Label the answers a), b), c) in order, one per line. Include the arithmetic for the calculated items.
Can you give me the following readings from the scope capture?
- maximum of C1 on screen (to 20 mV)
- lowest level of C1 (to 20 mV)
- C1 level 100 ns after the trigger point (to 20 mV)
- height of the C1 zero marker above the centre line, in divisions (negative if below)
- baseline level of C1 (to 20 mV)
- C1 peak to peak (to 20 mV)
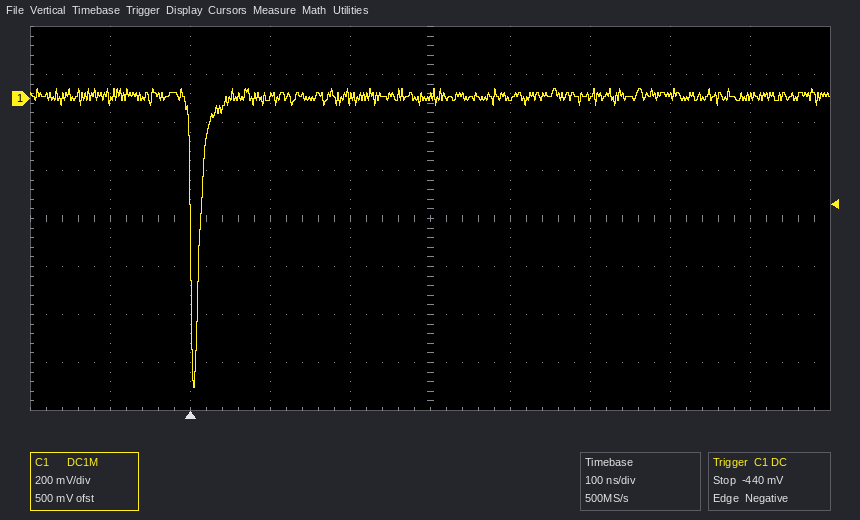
a) 40 mV
b) -1.20 V
c) 0 mV
d) +2.5 div
e) 0 mV
f) 40 mV − (-1.20 V) = 1.24 V
